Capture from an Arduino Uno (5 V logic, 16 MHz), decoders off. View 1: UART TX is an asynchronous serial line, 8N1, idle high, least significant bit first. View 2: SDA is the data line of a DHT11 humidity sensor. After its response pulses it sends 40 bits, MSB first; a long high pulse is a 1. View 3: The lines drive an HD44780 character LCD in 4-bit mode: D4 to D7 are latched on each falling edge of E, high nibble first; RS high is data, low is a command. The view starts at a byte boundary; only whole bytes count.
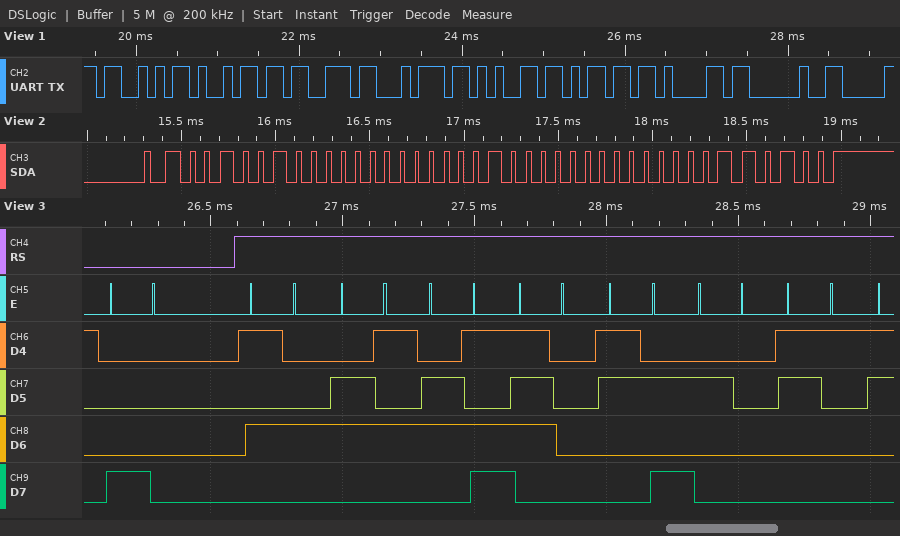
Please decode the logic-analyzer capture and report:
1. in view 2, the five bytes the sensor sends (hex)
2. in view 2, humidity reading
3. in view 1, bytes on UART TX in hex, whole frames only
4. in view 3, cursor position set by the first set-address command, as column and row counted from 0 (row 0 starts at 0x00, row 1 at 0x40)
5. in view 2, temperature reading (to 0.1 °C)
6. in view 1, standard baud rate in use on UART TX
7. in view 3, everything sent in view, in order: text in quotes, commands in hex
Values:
24 00 10 00 34
36 %
53 69 73 74 65 6D 61 20
column 0, row 0
16.0 °C
9600 baud
0x80 "Temp: 1"
